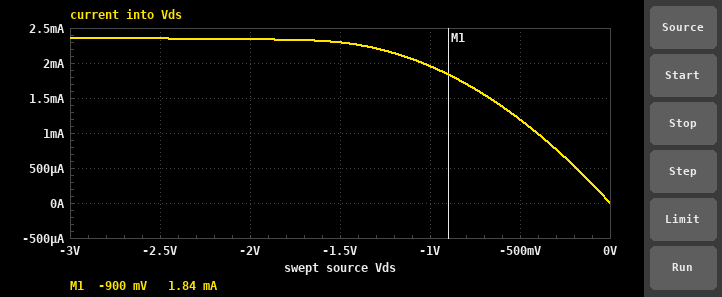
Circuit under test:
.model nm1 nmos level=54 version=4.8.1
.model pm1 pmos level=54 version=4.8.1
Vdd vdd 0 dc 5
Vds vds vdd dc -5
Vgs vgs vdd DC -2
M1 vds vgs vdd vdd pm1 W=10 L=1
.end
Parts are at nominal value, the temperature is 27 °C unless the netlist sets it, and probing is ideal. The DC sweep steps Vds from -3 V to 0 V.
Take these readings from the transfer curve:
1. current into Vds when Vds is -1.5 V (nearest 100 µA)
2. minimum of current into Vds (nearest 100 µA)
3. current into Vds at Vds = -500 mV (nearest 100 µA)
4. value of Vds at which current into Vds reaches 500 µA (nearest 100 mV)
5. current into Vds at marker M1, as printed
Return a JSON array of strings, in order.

["2.3 mA", "0 A", "1.2 mA", "-200 mV", "1.84 mA"]
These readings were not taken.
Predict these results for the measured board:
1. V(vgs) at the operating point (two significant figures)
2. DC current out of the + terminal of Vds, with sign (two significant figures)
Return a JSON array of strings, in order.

["3.0 V", "-2.4 mA"]
